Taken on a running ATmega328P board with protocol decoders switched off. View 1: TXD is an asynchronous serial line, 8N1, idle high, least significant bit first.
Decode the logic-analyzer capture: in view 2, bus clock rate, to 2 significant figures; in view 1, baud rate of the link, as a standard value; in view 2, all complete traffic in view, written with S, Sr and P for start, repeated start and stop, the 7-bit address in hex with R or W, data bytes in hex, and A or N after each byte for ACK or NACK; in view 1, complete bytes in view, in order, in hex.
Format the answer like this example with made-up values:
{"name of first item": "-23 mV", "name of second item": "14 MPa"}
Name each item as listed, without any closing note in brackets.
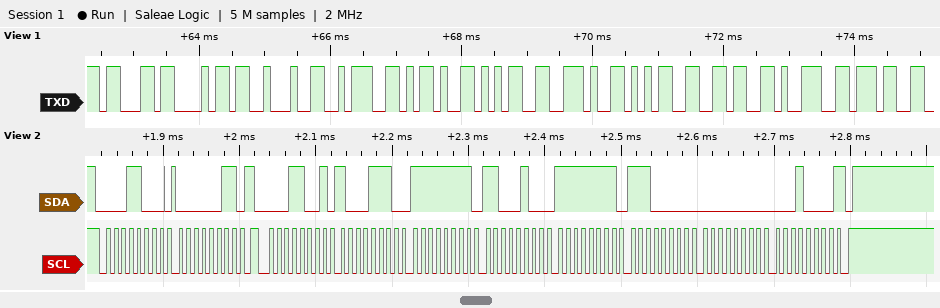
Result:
{"in view 2, bus clock rate, to 2 significant figures": "100 kHz", "in view 1, baud rate of the link, as a standard value": "9600 baud", "in view 2, all complete traffic in view, written with S, Sr and P for start, repeated start and stop, the 7-bit address in hex with R or W, data bytes in hex, and A or N after each byte for ACK or NACK": "S 0CW A 03 A Sr 0CR A 8E A FF A C4 A FF A E0 A 00 A 10 N P", "in view 1, complete bytes in view, in order, in hex": "63 68 22 3A 2D 35 2E 35 36 39 37"}
